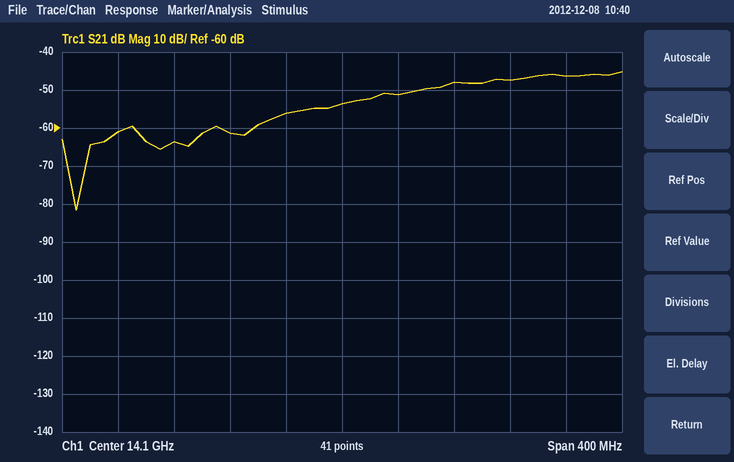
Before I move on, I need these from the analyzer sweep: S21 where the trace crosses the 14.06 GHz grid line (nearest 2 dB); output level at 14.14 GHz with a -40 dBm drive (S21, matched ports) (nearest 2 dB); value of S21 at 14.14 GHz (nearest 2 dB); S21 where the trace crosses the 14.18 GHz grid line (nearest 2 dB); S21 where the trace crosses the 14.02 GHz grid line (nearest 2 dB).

-56 dB
-92 dBm
-52 dB
-48 dB
-62 dB
